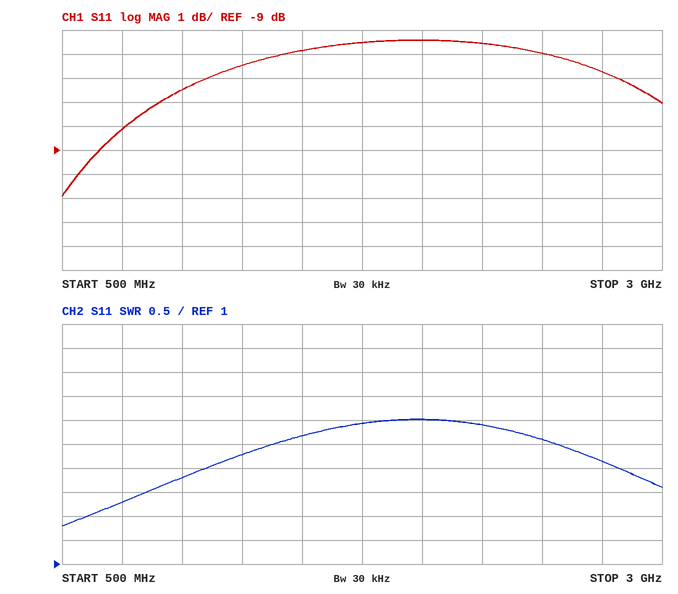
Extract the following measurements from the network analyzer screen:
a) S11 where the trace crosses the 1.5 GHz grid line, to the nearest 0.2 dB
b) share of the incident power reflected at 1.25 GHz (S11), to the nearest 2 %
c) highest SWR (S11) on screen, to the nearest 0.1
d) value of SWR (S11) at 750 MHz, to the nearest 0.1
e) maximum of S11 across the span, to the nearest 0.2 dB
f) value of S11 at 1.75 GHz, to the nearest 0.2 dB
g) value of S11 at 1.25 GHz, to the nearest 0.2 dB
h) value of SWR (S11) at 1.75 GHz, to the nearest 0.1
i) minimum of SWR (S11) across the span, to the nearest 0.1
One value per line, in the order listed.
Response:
-4.8 dB
28 %
4.0
2.3
-4.4 dB
-4.6 dB
-5.4 dB
3.9
1.8
